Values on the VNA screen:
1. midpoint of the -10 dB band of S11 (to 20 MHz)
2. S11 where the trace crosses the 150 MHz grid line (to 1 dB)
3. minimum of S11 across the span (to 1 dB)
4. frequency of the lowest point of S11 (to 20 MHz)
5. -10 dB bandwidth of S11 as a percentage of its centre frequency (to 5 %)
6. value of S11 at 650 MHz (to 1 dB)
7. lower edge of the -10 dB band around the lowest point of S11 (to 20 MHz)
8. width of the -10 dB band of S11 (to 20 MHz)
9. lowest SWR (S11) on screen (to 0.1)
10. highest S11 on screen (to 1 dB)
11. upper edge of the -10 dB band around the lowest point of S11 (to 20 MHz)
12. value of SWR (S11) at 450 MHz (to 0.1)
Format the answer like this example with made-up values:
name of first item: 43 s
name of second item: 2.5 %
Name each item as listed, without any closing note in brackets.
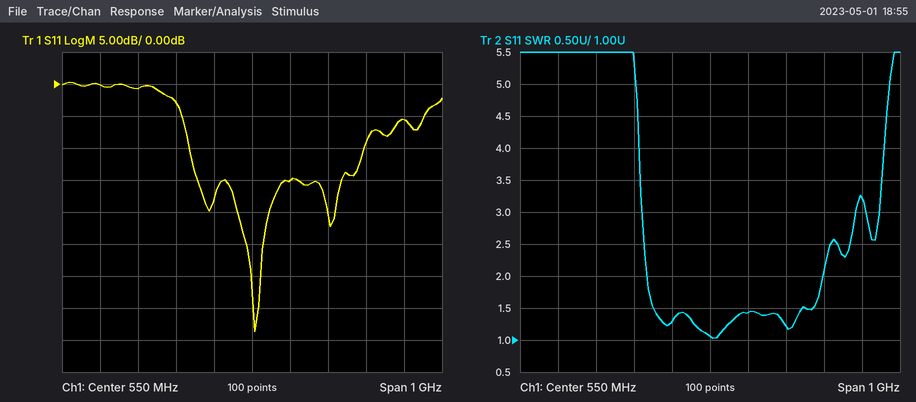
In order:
midpoint of the -10 dB band of S11: 620 MHz
S11 where the trace crosses the 150 MHz grid line: 0 dB
minimum of S11 across the span: -39 dB
frequency of the lowest point of S11: 560 MHz
-10 dB bandwidth of S11 as a percentage of its centre frequency: 75 %
value of S11 at 650 MHz: -15 dB
lower edge of the -10 dB band around the lowest point of S11: 380 MHz
width of the -10 dB band of S11: 460 MHz
lowest SWR (S11) on screen: 1.0
highest S11 on screen: 0 dB
upper edge of the -10 dB band around the lowest point of S11: 840 MHz
value of SWR (S11) at 450 MHz: 1.3
